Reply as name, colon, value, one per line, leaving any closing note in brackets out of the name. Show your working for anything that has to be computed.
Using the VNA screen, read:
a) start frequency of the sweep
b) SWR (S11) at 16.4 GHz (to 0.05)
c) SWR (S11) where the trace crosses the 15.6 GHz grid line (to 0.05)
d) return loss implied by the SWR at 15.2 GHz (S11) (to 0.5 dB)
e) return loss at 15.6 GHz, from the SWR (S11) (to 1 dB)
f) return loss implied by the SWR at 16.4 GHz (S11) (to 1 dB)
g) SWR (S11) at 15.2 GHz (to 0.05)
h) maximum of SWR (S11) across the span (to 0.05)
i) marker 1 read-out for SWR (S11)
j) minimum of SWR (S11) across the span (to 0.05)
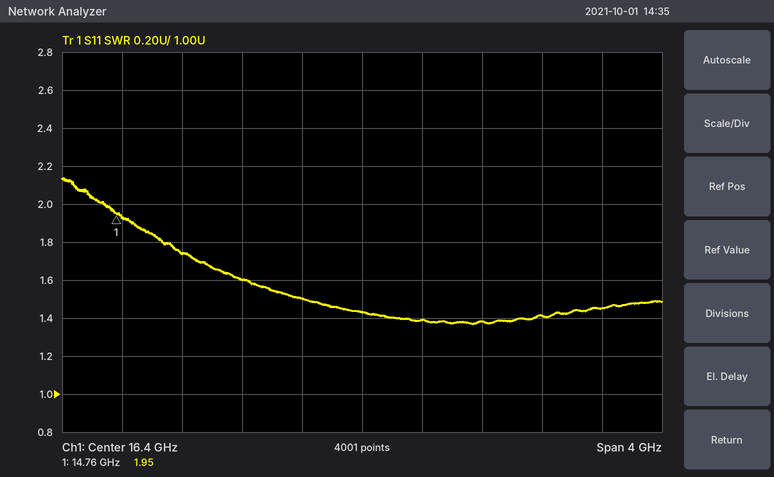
start frequency of the sweep: 14.4 GHz
SWR (S11) at 16.4 GHz: 1.45
SWR (S11) where the trace crosses the 15.6 GHz grid line: 1.60
return loss implied by the SWR at 15.2 GHz (S11): −20 log10((1.75 − 1)/(1.75 + 1)) ≈ 11.3 dB, so 11.5 dB to the nearest 0.5 dB
return loss at 15.6 GHz, from the SWR (S11): −20 log10((1.6 − 1)/(1.6 + 1)) ≈ 13 dB
return loss implied by the SWR at 16.4 GHz (S11): −20 log10((1.45 − 1)/(1.45 + 1)) ≈ 15 dB
SWR (S11) at 15.2 GHz: 1.75
maximum of SWR (S11) across the span: 2.15
marker 1 read-out for SWR: 1.95
minimum of SWR (S11) across the span: 1.35
